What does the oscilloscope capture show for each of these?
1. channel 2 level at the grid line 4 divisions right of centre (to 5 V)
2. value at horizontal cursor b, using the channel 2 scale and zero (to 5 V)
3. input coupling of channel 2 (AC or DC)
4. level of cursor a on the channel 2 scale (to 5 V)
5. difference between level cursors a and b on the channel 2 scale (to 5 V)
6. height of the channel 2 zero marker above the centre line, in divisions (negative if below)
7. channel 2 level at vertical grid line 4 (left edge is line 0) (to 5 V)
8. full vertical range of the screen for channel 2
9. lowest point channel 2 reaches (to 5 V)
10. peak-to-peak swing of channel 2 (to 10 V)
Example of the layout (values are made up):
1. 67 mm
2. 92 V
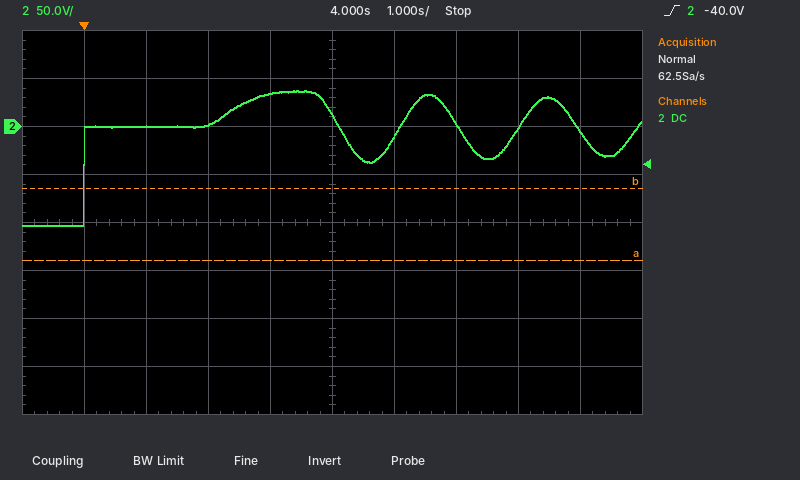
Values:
1. -5 V
2. -65 V
3. DC
4. -140 V
5. 75 V
6. +2.0 div
7. 35 V
8. 400 V
9. -105 V
10. 140 V
